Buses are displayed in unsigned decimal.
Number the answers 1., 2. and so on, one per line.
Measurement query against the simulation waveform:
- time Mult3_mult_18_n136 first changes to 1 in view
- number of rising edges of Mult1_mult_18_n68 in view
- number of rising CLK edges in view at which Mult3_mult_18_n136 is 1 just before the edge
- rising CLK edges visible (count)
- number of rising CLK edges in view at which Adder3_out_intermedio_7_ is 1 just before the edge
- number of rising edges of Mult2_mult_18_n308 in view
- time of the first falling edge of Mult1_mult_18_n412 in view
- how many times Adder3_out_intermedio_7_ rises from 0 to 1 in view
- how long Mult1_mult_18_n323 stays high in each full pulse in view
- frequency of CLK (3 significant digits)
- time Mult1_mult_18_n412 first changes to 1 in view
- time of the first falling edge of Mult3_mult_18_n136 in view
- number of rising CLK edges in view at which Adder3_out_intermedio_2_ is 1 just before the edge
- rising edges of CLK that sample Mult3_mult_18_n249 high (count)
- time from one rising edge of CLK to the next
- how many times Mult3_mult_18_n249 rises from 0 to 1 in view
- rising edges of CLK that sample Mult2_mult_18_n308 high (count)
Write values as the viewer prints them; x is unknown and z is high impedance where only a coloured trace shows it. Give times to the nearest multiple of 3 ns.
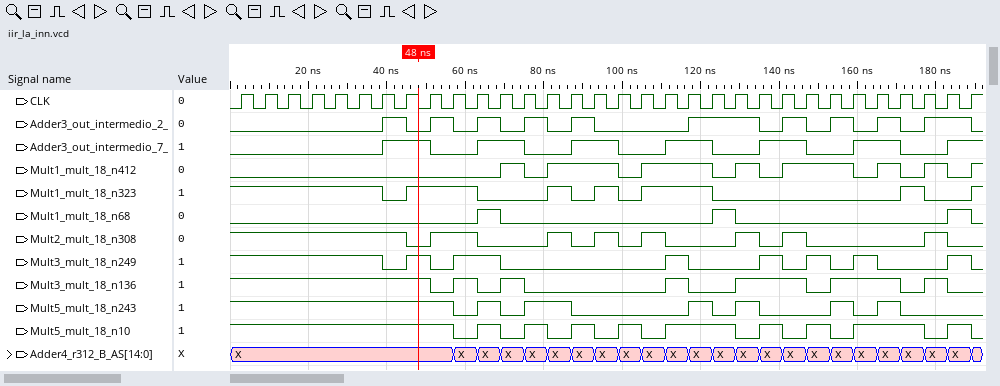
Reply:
1. 57 ns
2. 3
3. 19
4. 32
5. 13
6. 7
7. 75 ns
8. 7
9. 18 ns, 6 ns, 6 ns, 18 ns, 6 ns
10. 167 MHz
11. 69 ns
12. 51 ns
13. 13
14. 15
15. 6 ns
16. 7
17. 16
